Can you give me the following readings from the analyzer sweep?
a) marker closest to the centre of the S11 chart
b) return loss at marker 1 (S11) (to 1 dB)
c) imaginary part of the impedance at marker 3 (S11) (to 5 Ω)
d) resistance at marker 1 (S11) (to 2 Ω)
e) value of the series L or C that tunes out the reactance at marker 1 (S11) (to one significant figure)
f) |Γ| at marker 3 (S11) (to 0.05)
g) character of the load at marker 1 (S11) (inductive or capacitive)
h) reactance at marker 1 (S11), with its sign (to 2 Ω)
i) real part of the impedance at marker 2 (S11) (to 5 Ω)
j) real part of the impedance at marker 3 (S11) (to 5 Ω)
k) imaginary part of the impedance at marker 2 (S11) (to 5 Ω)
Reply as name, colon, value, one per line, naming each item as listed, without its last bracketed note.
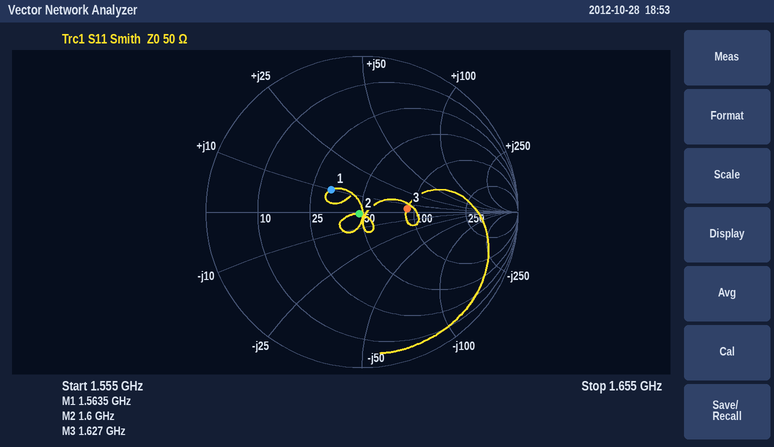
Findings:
marker closest to the centre of the S11 chart: marker 2
return loss at marker 1 (S11): 12 dB
imaginary part of the impedance at marker 3 (S11): +5 Ω
resistance at marker 1 (S11): 32 Ω
value of the series L or C that tunes out the reactance at marker 1 (S11): 10 pF
|Γ| at marker 3 (S11): 0.30
character of the load at marker 1 (S11): inductive
reactance at marker 1 (S11), with its sign: +10 Ω
real part of the impedance at marker 2 (S11): 50 Ω
real part of the impedance at marker 3 (S11): 90 Ω
imaginary part of the impedance at marker 2 (S11): 0 Ω
